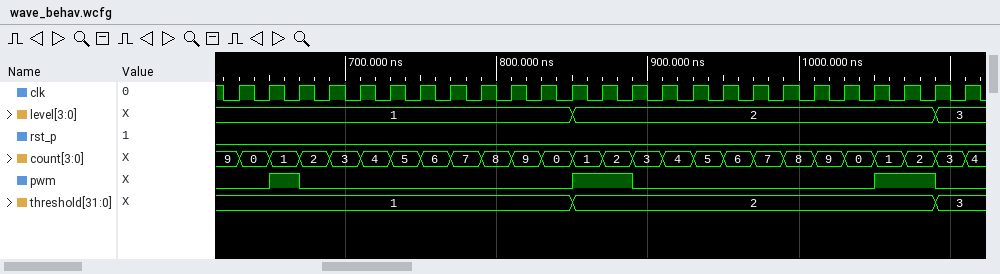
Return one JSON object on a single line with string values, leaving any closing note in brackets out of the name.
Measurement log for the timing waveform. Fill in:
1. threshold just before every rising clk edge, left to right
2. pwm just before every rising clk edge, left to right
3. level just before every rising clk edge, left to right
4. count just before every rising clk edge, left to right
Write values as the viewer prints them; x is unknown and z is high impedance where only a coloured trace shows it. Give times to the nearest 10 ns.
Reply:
{"threshold just before every rising clk edge, left to right": "1, 1, 1, 1, 1, 1, 1, 1, 1, 1, 1, 1, 2, 2, 2, 2, 2, 2, 2, 2, 2, 2, 2, 2, 3", "pwm just before every rising clk edge, left to right": "0 0 1 0 0 0 0 0 0 0 0 0 1 1 0 0 0 0 0 0 0 0 1 1 0", "level just before every rising clk edge, left to right": "1, 1, 1, 1, 1, 1, 1, 1, 1, 1, 1, 1, 2, 2, 2, 2, 2, 2, 2, 2, 2, 2, 2, 2, 3", "count just before every rising clk edge, left to right": "9, 0, 1, 2, 3, 4, 5, 6, 7, 8, 9, 0, 1, 2, 3, 4, 5, 6, 7, 8, 9, 0, 1, 2, 3"}
